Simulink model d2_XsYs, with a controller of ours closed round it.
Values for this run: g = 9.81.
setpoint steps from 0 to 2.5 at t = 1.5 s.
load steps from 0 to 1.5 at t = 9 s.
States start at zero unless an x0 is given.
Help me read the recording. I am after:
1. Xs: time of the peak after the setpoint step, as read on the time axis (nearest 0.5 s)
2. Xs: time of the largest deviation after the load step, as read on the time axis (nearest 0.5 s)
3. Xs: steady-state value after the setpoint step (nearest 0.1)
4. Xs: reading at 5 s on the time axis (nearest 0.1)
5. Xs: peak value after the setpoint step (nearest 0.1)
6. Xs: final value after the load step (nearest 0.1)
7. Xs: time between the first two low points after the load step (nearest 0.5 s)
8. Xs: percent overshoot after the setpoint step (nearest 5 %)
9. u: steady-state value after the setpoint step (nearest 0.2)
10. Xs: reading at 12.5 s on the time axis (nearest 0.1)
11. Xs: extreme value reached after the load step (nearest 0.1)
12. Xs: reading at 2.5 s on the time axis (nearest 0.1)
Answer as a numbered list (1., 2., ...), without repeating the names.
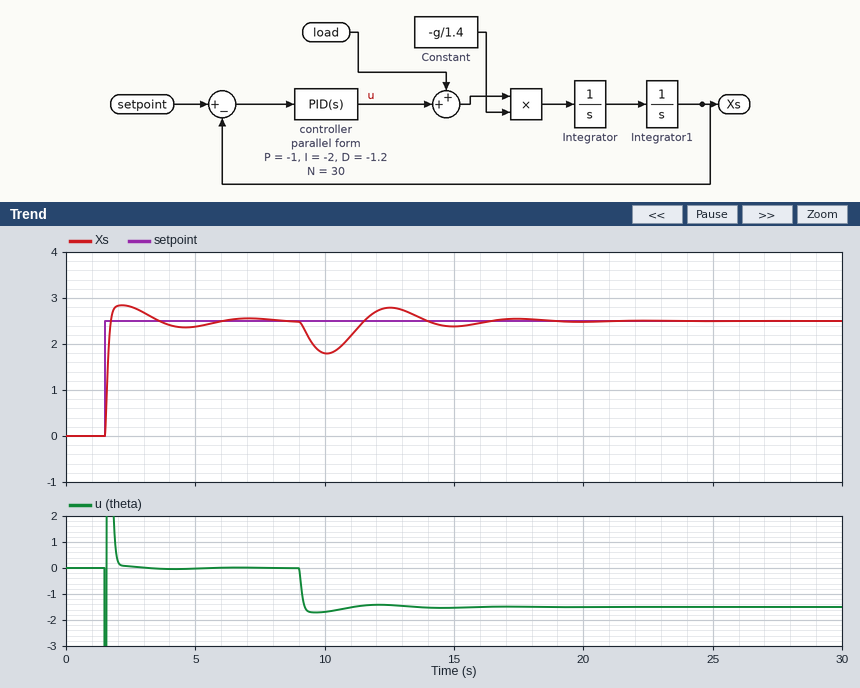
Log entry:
1. 2.0 s
2. 10.0 s
3. 2.5
4. 2.4
5. 2.8
6. 2.5
7. 5.0 s
8. 15 %
9. 0.0
10. 2.8
11. 1.8
12. 2.8
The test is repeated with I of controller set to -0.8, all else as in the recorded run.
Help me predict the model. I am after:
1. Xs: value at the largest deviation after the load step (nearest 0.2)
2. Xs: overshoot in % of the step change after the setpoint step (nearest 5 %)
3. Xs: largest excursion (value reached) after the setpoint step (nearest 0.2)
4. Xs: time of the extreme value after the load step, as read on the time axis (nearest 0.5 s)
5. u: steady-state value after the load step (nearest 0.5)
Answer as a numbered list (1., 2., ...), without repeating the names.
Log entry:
1. 1.6
2. 10 %
3. 2.8
4. 10.5 s
5. -1.5
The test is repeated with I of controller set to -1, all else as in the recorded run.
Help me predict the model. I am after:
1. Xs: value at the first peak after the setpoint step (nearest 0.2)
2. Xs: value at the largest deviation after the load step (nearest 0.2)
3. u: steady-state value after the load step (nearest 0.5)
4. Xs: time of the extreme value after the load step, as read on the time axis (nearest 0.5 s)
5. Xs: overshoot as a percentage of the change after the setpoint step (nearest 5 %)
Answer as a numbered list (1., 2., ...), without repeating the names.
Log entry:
1. 2.8
2. 1.6
3. -1.5
4. 10.5 s
5. 10 %
